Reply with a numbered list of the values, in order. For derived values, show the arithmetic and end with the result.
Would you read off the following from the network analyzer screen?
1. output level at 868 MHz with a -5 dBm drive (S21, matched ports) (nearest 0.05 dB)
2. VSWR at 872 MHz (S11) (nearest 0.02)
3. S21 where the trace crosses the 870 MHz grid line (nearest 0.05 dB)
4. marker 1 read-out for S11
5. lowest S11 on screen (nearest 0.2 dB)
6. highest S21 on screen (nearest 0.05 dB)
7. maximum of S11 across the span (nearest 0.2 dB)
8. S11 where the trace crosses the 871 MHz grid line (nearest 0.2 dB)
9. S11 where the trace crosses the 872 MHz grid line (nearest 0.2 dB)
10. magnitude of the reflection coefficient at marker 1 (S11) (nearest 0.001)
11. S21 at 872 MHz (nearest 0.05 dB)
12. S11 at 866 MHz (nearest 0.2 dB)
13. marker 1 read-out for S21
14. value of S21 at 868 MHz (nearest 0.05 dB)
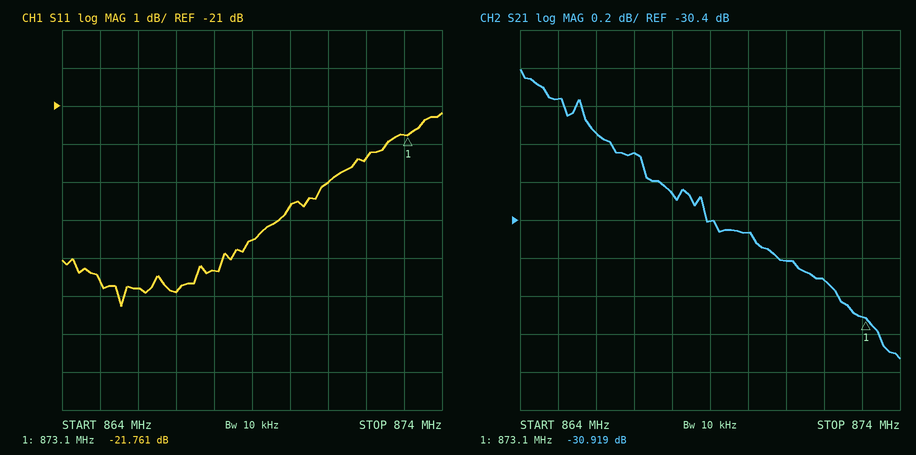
1. -5 dBm + (-30.25 dB) = -35.25 dBm
2. |Γ| = 10^(-22.4/20) = 0.0759; VSWR = (1 + 0.0759)/(1 − 0.0759) ≈ 1.16
3. -30.45 dB
4. -21.761 dB
5. -26.2 dB
6. -29.60 dB
7. -21.2 dB
8. -23.0 dB
9. -22.4 dB
10. 10^(-21.761/20) ≈ 0.082
11. -30.70 dB
12. -25.8 dB
13. -30.919 dB
14. -30.25 dB
